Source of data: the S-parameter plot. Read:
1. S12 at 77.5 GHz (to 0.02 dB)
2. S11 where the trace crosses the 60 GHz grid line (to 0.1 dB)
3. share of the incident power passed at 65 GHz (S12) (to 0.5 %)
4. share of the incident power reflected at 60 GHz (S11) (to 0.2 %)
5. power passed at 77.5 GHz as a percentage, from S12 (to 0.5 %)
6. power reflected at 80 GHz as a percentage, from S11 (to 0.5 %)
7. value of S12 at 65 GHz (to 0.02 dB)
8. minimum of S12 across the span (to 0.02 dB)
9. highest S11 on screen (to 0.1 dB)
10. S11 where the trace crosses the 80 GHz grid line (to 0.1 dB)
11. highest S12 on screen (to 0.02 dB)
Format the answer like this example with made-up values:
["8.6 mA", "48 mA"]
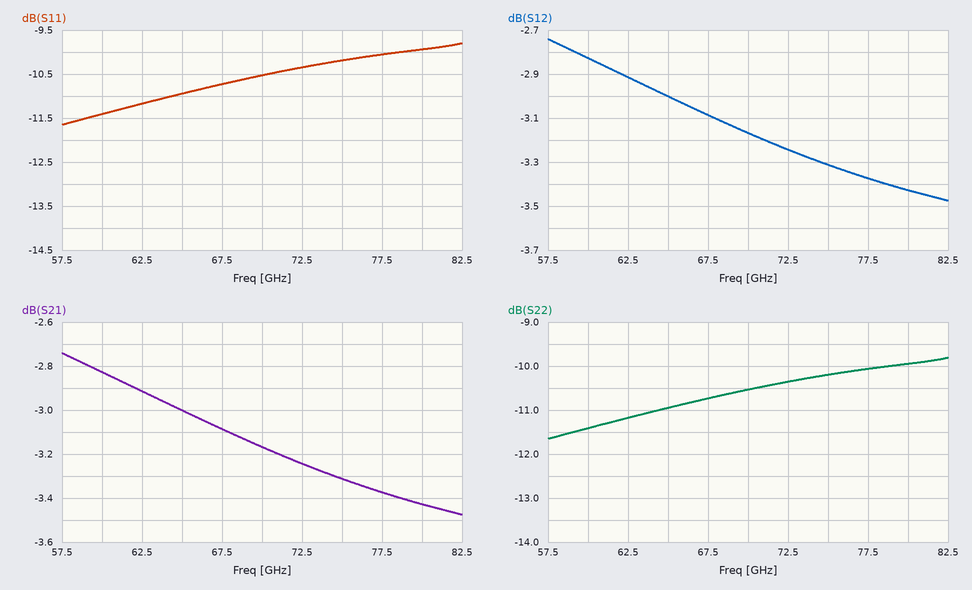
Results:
["-3.38 dB", "-11.4 dB", "50.0 %", "7.2 %", "46.0 %", "10.0 %", "-3.00 dB", "-3.48 dB", "-9.8 dB", "-9.9 dB", "-2.74 dB"]
